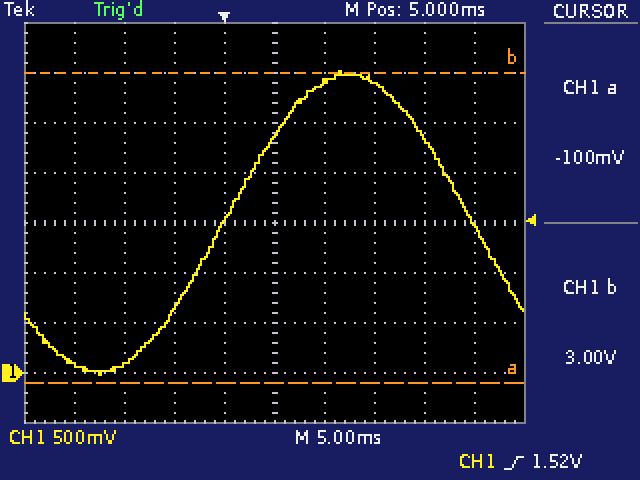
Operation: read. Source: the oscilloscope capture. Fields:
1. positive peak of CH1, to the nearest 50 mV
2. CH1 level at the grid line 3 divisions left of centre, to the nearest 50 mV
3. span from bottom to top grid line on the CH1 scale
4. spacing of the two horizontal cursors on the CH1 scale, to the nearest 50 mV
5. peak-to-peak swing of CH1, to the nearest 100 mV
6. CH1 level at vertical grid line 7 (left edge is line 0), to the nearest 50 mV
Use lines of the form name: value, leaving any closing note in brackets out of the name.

positive peak of CH1, to the nearest 50 mV: 3.00 V
CH1 level at the grid line 3 divisions left of centre, to the nearest 50 mV: 100 mV
span from bottom to top grid line on the CH1 scale: 4 V
spacing of the two horizontal cursors on the CH1 scale, to the nearest 50 mV: 3.10 V
peak-to-peak swing of CH1, to the nearest 100 mV: 3.00 V
CH1 level at vertical grid line 7 (left edge is line 0), to the nearest 50 mV: 2.90 V
